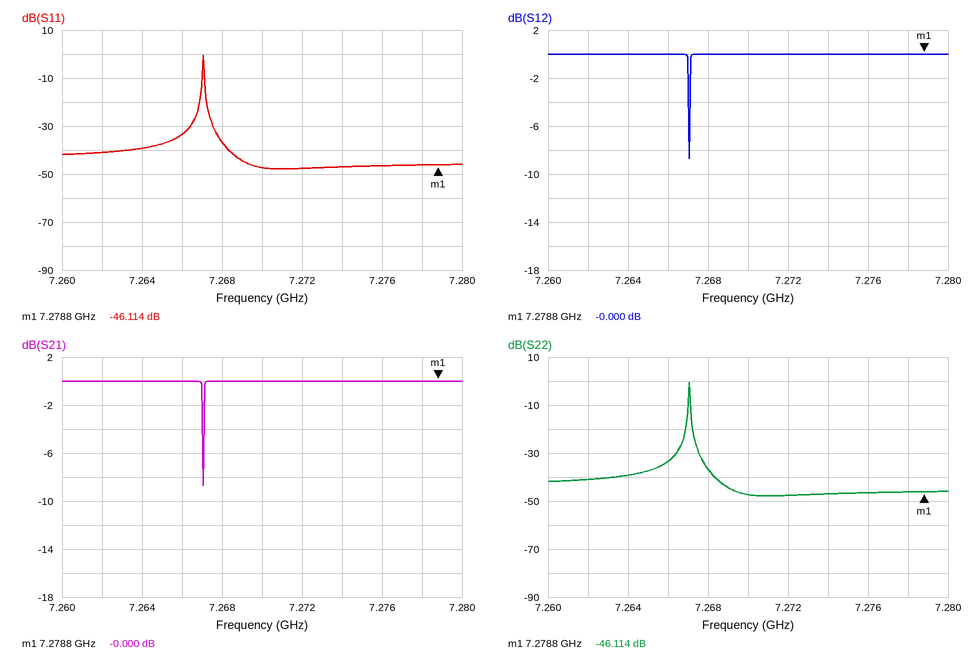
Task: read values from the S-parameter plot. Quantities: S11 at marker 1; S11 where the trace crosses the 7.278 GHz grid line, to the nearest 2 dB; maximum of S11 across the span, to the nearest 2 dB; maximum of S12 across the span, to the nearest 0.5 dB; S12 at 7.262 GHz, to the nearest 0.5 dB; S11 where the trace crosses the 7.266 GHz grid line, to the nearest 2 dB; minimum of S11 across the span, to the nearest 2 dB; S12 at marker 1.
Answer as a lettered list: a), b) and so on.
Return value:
a) -46.114 dB
b) -46 dB
c) 0 dB
d) 0.0 dB
e) 0.0 dB
f) -34 dB
g) -48 dB
h) -0.000 dB
